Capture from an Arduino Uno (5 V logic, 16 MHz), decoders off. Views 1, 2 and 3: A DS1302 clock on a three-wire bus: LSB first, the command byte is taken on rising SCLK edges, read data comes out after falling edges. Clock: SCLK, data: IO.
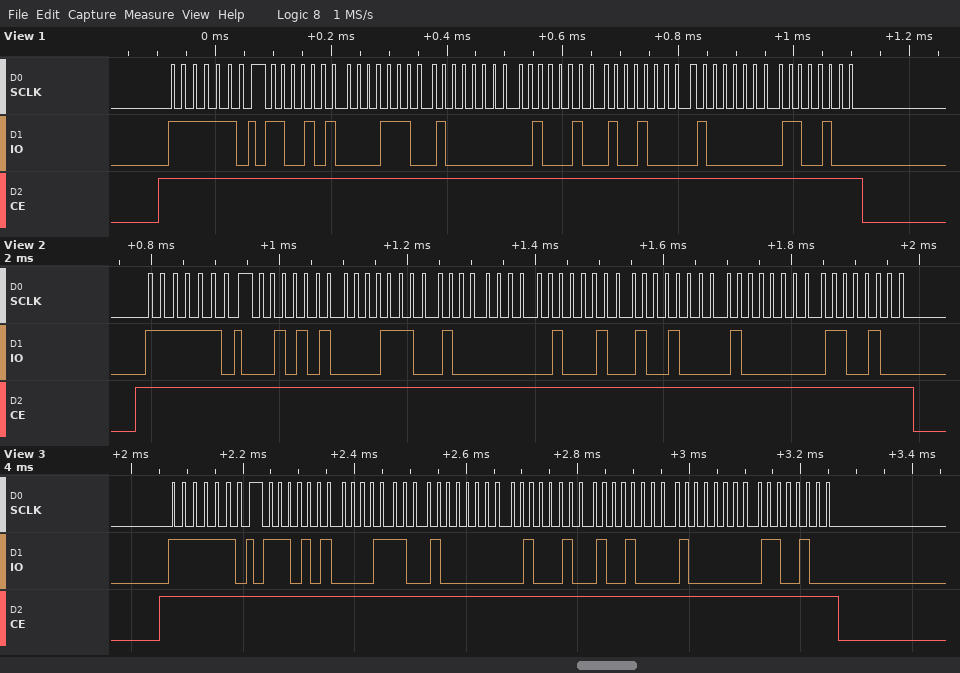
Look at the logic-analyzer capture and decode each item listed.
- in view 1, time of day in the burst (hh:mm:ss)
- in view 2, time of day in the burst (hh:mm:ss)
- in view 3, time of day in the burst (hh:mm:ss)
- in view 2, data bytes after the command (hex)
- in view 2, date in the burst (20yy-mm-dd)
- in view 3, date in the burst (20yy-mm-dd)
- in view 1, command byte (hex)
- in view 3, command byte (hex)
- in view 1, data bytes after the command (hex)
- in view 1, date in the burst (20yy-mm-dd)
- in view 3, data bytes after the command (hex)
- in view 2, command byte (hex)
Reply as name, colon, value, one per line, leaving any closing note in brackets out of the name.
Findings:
in view 1, time of day in the burst: 01:38:53
in view 2, time of day in the burst: 01:38:54
in view 3, time of day in the burst: 01:38:57
in view 2, data bytes after the command: 54 38 01 22 09 01 13
in view 2, date in the burst: 2013-09-22
in view 3, date in the burst: 2013-09-22
in view 1, command byte: 0xBF
in view 3, command byte: 0xBF
in view 1, data bytes after the command: 53 38 01 22 09 01 13
in view 1, date in the burst: 2013-09-22
in view 3, data bytes after the command: 57 38 01 22 09 01 13
in view 2, command byte: 0xBF
